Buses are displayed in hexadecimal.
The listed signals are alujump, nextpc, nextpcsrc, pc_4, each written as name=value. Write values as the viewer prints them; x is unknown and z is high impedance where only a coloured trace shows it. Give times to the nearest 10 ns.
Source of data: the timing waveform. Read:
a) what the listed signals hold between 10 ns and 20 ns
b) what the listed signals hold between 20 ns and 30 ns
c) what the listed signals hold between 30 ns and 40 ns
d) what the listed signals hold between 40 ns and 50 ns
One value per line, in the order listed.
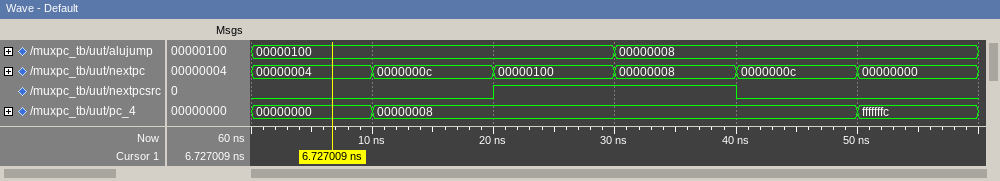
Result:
alujump=00000100, nextpc=0000000c, nextpcsrc=0, pc_4=00000008
alujump=00000100, nextpc=00000100, nextpcsrc=1, pc_4=00000008
alujump=00000008, nextpc=00000008, nextpcsrc=1, pc_4=00000008
alujump=00000008, nextpc=0000000c, nextpcsrc=0, pc_4=00000008
